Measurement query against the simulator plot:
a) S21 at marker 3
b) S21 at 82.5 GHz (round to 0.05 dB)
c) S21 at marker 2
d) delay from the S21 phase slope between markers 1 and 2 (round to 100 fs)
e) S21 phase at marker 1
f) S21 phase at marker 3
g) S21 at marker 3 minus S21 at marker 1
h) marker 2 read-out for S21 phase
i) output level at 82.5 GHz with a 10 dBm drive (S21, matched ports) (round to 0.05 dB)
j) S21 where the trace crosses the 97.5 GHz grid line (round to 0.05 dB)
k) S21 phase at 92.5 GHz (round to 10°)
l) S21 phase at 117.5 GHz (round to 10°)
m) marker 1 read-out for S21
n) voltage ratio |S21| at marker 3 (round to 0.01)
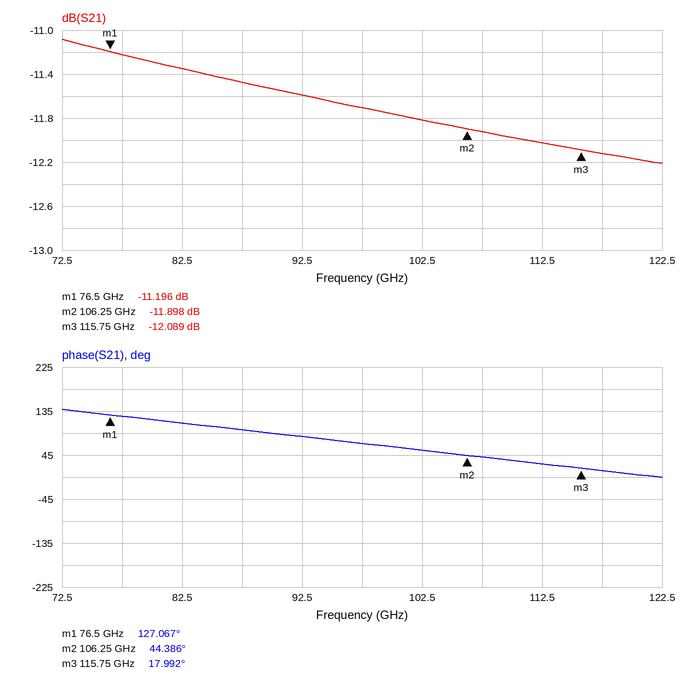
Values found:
-12.089 dB
-11.35 dB
-11.898 dB
7.7 ps
127.067°
17.992°
-0.893 dB
44.386°
-1.35 dBm
-11.70 dB
80°
10°
-11.196 dB
0.25
